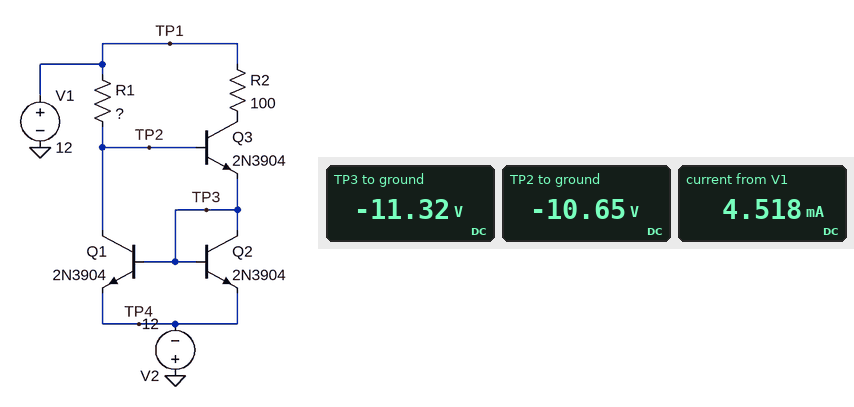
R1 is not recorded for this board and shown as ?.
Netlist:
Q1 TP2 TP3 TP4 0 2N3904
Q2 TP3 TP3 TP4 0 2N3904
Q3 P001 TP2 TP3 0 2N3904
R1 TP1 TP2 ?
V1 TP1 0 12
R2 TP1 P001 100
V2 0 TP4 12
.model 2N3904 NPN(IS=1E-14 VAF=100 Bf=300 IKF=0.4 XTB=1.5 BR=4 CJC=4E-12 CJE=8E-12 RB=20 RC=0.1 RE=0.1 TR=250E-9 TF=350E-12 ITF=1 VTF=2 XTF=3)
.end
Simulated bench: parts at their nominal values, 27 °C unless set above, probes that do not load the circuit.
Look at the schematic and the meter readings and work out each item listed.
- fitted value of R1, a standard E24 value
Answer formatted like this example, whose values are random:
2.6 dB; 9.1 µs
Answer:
10 kΩ
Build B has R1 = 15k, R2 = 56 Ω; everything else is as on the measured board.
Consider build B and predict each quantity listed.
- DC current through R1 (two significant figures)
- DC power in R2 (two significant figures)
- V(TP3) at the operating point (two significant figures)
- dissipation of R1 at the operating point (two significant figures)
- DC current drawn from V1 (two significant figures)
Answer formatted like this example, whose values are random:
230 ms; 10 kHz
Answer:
1.5 mA; 130 µW; -11 V; 34 mW; 3.0 mA
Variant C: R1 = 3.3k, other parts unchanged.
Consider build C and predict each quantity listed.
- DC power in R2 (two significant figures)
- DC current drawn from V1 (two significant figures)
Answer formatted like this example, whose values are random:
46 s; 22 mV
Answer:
4.6 mW; 14 mA
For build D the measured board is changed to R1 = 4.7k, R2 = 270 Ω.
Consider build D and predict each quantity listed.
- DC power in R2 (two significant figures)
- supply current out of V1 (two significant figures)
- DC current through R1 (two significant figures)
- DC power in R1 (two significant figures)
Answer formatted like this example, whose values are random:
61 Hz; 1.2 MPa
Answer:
6.2 mW; 9.6 mA; 4.8 mA; 110 mW
